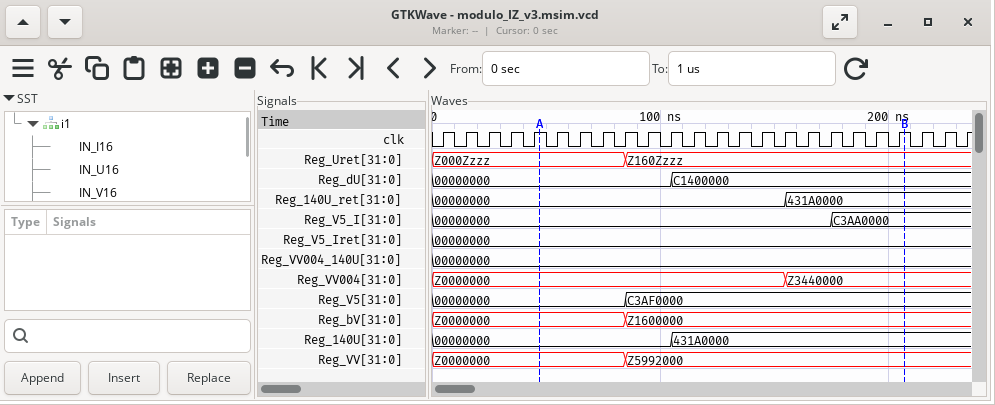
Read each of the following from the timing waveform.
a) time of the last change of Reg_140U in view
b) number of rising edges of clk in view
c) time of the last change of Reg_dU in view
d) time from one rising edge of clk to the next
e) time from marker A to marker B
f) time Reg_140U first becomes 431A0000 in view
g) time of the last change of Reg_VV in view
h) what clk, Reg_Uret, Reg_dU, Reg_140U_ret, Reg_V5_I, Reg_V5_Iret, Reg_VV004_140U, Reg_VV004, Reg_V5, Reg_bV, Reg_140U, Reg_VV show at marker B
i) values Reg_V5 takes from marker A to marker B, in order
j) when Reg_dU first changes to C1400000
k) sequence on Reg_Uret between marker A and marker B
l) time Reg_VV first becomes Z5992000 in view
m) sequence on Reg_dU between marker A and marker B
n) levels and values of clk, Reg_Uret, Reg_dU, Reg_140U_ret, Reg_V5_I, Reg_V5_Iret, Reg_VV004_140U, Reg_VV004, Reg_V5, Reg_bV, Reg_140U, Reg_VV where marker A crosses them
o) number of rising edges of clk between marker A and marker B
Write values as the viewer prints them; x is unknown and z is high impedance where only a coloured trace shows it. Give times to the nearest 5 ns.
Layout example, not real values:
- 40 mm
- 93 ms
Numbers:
- 105 ns
- 24
- 105 ns
- 10 ns
- 160 ns
- 105 ns
- 85 ns
- clk=1, Reg_Uret=Z160Zzzz, Reg_dU=C1400000, Reg_140U_ret=431A0000, Reg_V5_I=C3AA0000, Reg_V5_Iret=00000000, Reg_VV004_140U=00000000, Reg_VV004=Z3440000, Reg_V5=C3AF0000, Reg_bV=Z1600000, Reg_140U=431A0000, Reg_VV=Z5992000
- 00000000, C3AF0000
- 105 ns
- Z000Zzzz, Z160Zzzz
- 85 ns
- 00000000, C1400000
- clk=1, Reg_Uret=Z000Zzzz, Reg_dU=00000000, Reg_140U_ret=00000000, Reg_V5_I=00000000, Reg_V5_Iret=00000000, Reg_VV004_140U=00000000, Reg_VV004=Z0000000, Reg_V5=00000000, Reg_bV=Z0000000, Reg_140U=00000000, Reg_VV=Z0000000
- 16
